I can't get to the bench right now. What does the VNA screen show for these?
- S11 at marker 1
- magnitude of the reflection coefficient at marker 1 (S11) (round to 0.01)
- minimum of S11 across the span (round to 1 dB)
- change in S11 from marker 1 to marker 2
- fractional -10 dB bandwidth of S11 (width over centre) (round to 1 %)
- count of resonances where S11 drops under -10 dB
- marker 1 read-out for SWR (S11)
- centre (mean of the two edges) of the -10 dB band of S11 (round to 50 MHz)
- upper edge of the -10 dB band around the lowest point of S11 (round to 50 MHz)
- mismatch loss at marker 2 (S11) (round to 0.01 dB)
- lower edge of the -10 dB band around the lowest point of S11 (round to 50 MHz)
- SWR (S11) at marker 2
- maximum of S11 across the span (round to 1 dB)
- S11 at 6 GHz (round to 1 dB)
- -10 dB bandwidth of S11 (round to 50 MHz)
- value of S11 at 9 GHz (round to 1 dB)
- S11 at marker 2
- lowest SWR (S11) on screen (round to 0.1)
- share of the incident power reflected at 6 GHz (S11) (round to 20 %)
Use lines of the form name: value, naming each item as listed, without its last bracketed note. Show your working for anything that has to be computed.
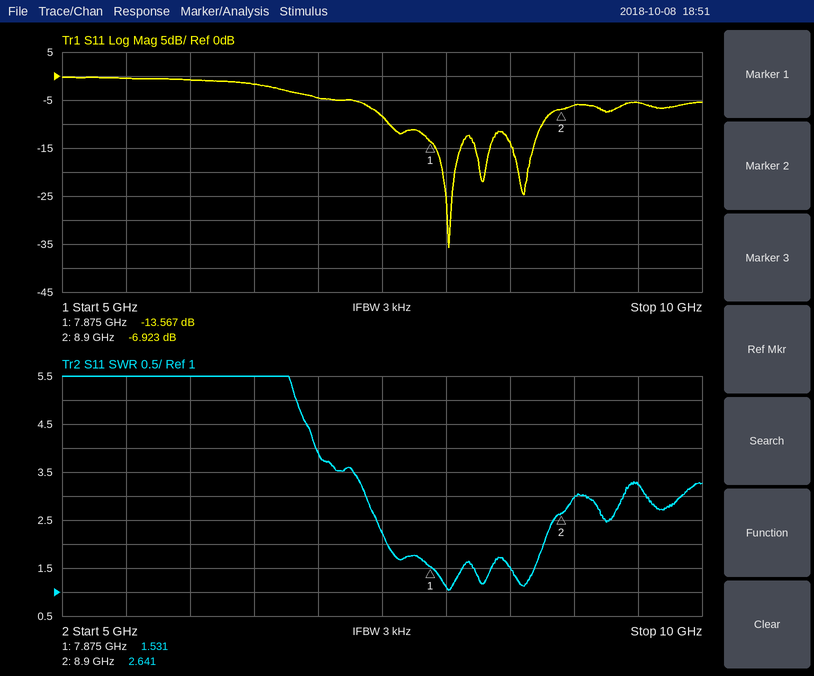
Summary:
S11 at marker 1: -13.567 dB
magnitude of the reflection coefficient at marker 1 (S11): 10^(-13.567/20) ≈ 0.21
minimum of S11 across the span: -36 dB
change in S11 from marker 1 to marker 2: -6.923 − (-13.567) = 6.644 dB
fractional -10 dB bandwidth of S11 (width over centre): 1.2 GHz / 8.15 GHz ≈ 15 %
count of resonances where S11 drops under -10 dB: 3
marker 1 read-out for SWR: 1.531
centre (mean of the two edges) of the -10 dB band of S11: 8.15 GHz
upper edge of the -10 dB band around the lowest point of S11: 8.75 GHz
mismatch loss at marker 2 (S11): −10 log10(1 − 10^(-6.923/10)) ≈ 0.99 dB
lower edge of the -10 dB band around the lowest point of S11: 7.55 GHz
SWR (S11) at marker 2: 2.641
maximum of S11 across the span: 0 dB
S11 at 6 GHz: -1 dB
-10 dB bandwidth of S11: 8.75 GHz − 7.55 GHz = 1.20 GHz
value of S11 at 9 GHz: -6 dB
S11 at marker 2: -6.923 dB
lowest SWR (S11) on screen: 1.0
share of the incident power reflected at 6 GHz (S11): 10^(-1/10) ≈ 79.4 %, so 80 % to the nearest 20 %
